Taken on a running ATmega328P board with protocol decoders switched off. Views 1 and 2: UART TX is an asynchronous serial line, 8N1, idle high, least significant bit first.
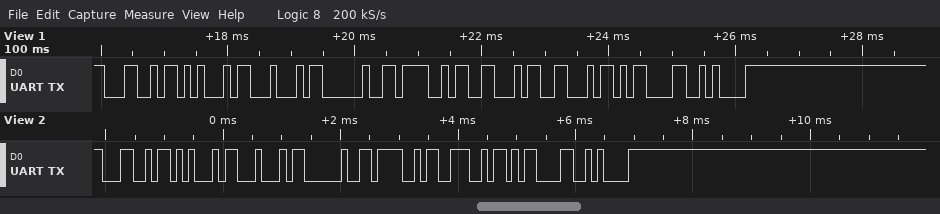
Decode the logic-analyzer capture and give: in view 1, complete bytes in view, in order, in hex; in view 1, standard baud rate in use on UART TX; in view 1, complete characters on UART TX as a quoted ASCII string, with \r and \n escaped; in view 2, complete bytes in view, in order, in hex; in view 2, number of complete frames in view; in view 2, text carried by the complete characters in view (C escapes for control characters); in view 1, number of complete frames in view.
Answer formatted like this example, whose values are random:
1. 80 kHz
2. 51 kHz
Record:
1. 4C 45 44 20 4F 46 46 0D 0A
2. 9600 baud
3. "LED OFF\r\n"
4. 4C 45 44 20 4F 4E 0D 0A
5. 8
6. "LED ON\r\n"
7. 9
